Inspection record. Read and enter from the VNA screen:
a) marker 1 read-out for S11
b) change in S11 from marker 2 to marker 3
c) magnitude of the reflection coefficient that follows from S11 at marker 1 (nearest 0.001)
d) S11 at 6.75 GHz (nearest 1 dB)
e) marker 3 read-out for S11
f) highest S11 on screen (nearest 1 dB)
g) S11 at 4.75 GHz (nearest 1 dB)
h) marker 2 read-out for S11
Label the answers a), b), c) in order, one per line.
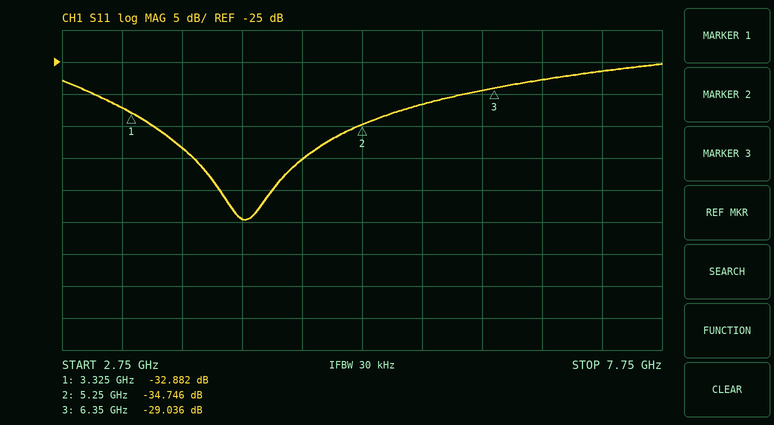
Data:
a) -32.882 dB
b) 5.710 dB
c) 0.023
d) -28 dB
e) -29.036 dB
f) -25 dB
g) -40 dB
h) -34.746 dB
